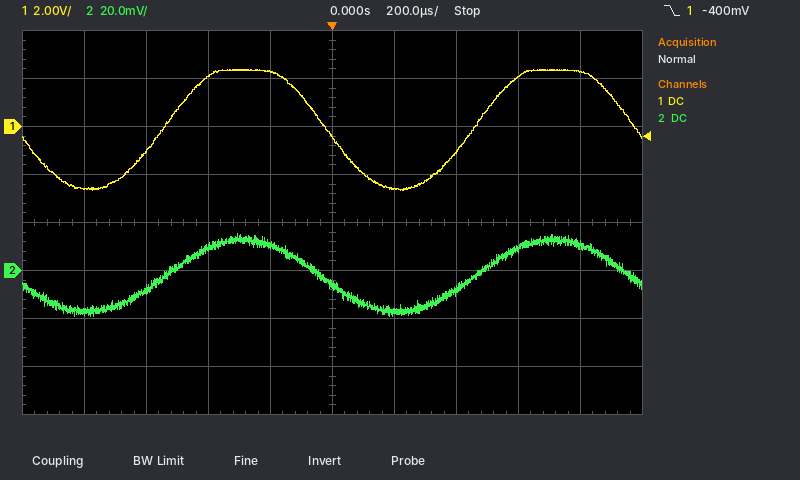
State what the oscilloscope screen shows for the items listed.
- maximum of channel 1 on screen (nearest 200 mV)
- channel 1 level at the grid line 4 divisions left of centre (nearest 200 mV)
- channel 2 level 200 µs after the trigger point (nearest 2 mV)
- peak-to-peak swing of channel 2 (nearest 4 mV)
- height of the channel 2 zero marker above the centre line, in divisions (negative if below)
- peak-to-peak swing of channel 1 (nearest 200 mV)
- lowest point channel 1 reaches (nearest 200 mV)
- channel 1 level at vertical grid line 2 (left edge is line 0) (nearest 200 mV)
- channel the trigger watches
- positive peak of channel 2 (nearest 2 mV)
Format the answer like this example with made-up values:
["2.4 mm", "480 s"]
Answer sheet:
["2.4 V", "-2.6 V", "-18 mV", "36 mV", "-1.0 div", "5.0 V", "-2.6 V", "-1.0 V", "channel 1", "16 mV"]
